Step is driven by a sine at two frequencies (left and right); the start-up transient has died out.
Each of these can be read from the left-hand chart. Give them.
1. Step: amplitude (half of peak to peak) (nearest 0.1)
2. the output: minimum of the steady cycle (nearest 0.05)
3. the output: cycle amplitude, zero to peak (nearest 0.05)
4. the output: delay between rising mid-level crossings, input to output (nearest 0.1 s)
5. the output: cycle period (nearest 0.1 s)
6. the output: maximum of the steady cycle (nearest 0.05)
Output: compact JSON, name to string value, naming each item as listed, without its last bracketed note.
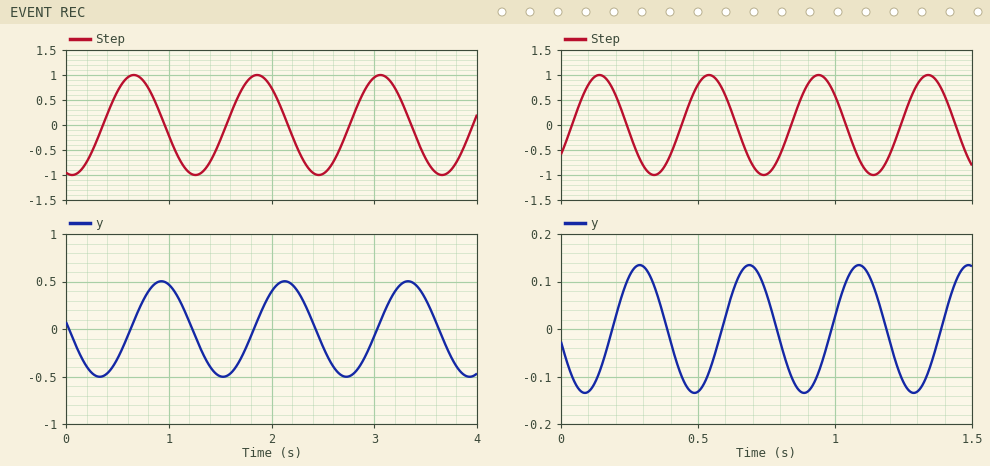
{"Step: amplitude (half of peak to peak)": "1.0", "the output: minimum of the steady cycle": "-0.50", "the output: cycle amplitude, zero to peak": "0.50", "the output: delay between rising mid-level crossings, input to output": "0.3 s", "the output: cycle period": "1.2 s", "the output: maximum of the steady cycle": "0.50"}
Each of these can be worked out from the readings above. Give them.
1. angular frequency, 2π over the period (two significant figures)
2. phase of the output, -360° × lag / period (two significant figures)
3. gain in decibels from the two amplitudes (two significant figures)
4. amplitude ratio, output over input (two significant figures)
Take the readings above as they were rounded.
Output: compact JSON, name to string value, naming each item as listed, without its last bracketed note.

{"angular frequency, 2π over the period": "5.2 rad/s", "phase of the output, -360° × lag / period": "-90°", "gain in decibels from the two amplitudes": "-6.0 dB", "amplitude ratio, output over input": "0.50"}
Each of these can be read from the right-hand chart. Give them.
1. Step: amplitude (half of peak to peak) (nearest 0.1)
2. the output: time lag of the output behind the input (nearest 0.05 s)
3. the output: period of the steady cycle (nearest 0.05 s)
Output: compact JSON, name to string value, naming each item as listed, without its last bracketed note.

{"Step: amplitude (half of peak to peak)": "1.0", "the output: time lag of the output behind the input": "0.15 s", "the output: period of the steady cycle": "0.40 s"}
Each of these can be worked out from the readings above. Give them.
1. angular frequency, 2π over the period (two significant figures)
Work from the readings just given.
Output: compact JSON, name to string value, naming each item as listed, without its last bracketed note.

{"angular frequency, 2π over the period": "16 rad/s"}
